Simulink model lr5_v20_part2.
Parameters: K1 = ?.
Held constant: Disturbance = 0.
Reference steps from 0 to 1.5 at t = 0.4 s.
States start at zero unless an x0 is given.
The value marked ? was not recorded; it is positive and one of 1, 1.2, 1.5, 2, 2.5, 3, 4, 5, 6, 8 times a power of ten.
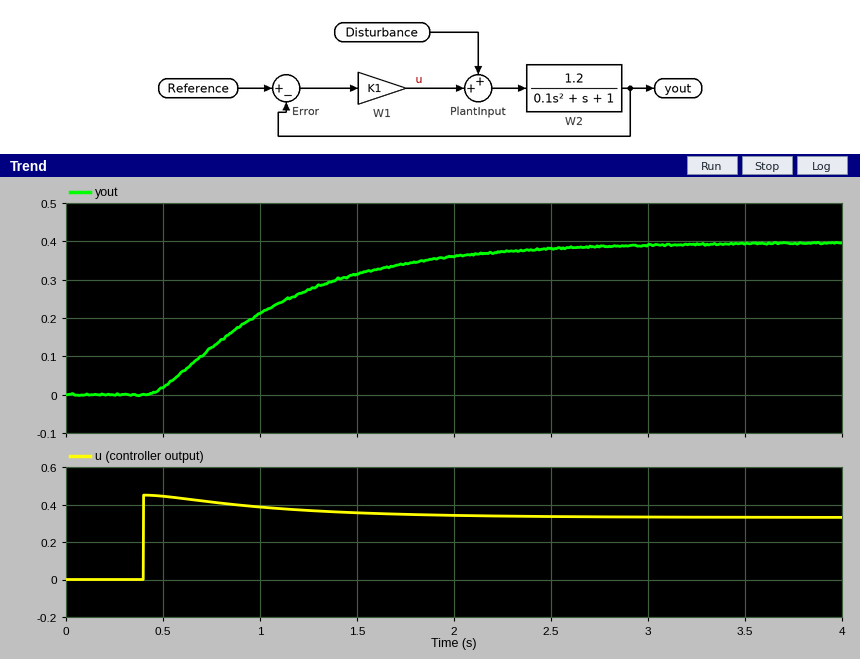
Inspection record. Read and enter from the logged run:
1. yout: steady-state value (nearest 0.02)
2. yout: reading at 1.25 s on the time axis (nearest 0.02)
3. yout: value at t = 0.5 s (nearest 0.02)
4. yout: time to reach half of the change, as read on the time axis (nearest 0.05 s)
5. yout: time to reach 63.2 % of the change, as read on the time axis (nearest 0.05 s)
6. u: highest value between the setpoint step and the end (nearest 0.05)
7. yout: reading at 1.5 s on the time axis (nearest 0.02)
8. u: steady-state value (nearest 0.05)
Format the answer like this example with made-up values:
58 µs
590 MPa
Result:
0.40
0.28
0.02
0.95 s
1.15 s
0.45
0.32
0.35
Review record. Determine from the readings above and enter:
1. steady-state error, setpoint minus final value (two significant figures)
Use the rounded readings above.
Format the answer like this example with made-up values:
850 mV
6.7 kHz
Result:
1.1
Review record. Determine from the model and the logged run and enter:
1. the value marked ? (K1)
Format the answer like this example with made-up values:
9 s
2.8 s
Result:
0.3
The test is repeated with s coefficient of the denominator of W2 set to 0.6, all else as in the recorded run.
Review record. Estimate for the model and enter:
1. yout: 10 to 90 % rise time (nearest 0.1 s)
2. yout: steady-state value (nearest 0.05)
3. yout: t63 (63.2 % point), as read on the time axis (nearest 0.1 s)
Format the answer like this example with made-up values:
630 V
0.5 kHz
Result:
0.7 s
0.40
0.9 s
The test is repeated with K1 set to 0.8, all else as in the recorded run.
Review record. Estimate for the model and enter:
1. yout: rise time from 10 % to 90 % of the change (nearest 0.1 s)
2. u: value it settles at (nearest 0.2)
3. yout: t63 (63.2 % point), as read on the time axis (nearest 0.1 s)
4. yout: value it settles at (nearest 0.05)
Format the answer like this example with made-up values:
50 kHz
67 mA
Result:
0.9 s
0.6
0.9 s
0.75
